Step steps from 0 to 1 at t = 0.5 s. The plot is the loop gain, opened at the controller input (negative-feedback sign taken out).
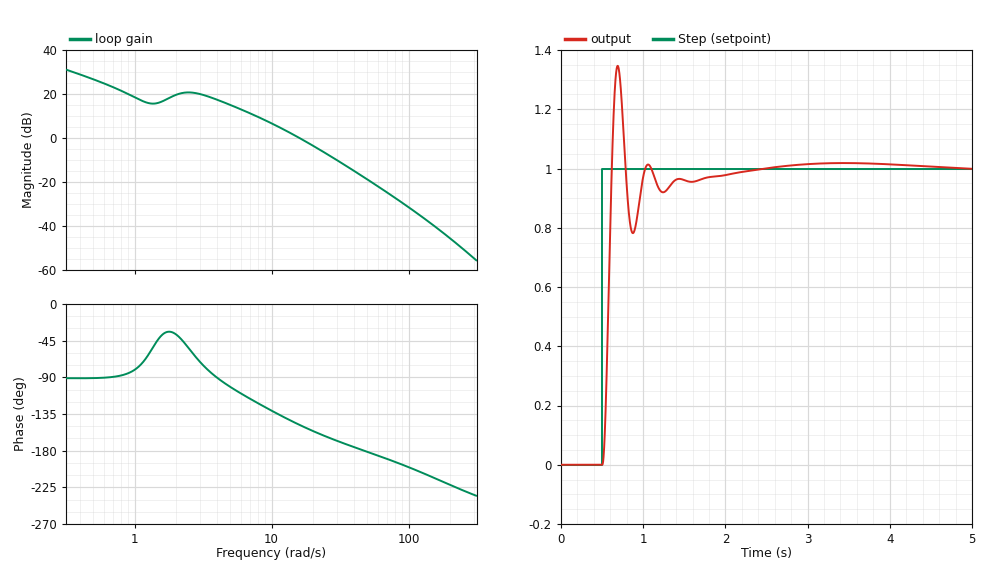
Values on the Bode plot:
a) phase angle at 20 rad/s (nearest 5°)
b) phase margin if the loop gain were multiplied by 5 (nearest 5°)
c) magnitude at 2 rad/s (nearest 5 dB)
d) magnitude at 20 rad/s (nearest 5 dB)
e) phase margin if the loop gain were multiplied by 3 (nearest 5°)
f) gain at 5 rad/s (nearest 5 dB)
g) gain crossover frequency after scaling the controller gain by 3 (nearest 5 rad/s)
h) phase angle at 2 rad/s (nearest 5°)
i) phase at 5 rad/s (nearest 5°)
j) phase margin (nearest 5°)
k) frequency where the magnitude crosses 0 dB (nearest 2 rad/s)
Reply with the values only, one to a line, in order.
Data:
-155°
5°
20 dB
-5 dB
15°
15 dB
30 rad/s
-35°
-100°
30°
16 rad/s
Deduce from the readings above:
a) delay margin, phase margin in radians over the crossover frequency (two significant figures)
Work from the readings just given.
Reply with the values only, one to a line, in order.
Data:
0.033 s
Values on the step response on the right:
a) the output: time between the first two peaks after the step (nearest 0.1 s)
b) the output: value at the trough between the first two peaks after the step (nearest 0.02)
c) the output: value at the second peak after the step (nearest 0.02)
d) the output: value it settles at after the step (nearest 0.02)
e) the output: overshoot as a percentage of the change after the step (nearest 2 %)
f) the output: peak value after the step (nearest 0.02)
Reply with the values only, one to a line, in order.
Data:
0.4 s
0.78
1.02
1.00
34 %
1.34
